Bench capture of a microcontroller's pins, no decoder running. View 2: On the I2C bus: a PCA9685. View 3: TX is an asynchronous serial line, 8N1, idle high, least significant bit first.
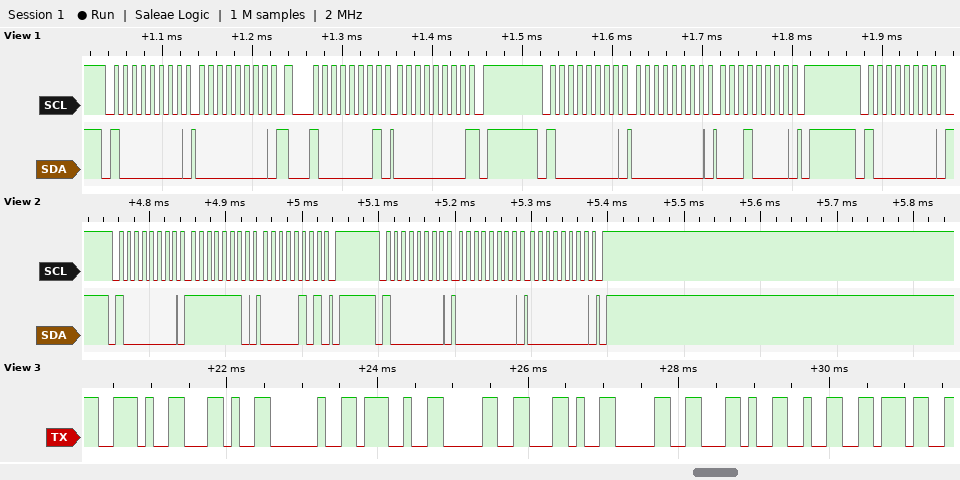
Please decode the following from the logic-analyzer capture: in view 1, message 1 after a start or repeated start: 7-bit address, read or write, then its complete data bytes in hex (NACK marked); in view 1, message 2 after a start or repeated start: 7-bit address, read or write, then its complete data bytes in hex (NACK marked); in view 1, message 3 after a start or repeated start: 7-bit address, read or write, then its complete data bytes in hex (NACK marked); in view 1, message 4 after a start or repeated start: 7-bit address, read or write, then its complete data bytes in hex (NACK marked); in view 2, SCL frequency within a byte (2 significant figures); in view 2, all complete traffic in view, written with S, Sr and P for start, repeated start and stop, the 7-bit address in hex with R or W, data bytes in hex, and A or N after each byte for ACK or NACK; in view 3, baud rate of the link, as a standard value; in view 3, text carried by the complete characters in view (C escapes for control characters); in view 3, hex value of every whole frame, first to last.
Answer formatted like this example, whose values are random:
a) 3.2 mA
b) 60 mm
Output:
a) 0x40 write: 00
b) 0x40 read: 00 NACK
c) 0x40 write: 00 10
d) 0x40 write
e) 100 kHz
f) S 40W A FE A 05 A P S 40W A 00 A 00 A P
g) 9600 baud
h) "., '0,0,27"
i) 2E 2C 20 27 30 2C 30 2C 32 37
